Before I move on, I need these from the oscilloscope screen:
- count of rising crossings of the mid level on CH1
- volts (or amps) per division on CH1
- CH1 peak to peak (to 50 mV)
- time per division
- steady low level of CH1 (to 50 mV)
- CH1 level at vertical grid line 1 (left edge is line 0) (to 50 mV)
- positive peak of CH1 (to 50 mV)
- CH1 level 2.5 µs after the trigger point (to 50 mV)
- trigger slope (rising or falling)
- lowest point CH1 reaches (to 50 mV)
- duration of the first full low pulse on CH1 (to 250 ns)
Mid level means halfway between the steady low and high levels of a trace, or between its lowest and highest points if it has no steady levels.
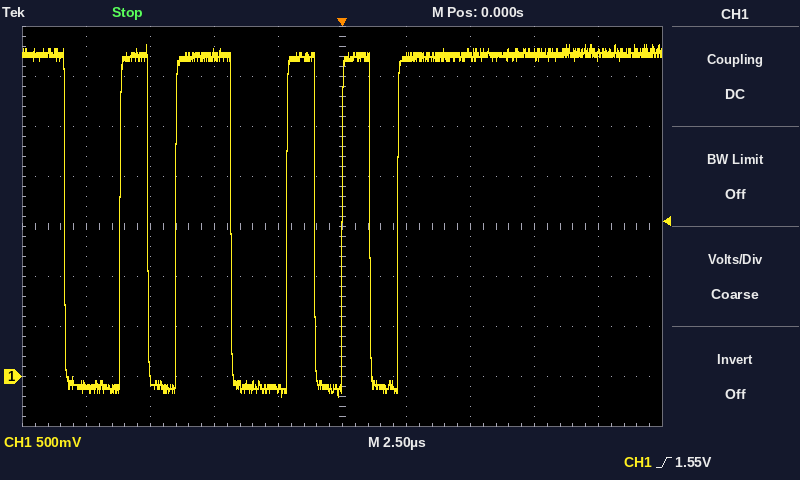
5
500 mV
3.50 V
2.5 µs
-100 mV
-100 mV
3.30 V
3.20 V
rising
-200 mV
2.25 µs
